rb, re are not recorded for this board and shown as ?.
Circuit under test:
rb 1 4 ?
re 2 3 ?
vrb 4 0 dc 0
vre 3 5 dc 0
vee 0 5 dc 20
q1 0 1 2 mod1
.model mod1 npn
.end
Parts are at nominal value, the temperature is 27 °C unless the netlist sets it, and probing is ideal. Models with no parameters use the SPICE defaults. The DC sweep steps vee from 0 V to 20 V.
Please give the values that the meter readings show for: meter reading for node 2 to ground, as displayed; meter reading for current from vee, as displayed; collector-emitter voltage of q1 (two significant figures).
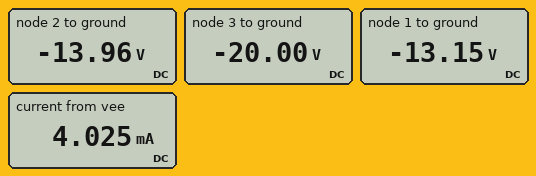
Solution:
-13.96 V
4.025 mA
14 V
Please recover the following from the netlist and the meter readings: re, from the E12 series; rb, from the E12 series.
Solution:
1.5 kΩ
330 kΩ
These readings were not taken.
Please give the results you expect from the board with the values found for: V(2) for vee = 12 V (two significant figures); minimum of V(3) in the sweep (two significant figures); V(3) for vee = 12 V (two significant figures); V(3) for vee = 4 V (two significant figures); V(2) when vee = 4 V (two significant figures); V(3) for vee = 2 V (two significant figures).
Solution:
-8.5 V
-20 V
-12 V
-4.0 V
-3.0 V
-2.0 V
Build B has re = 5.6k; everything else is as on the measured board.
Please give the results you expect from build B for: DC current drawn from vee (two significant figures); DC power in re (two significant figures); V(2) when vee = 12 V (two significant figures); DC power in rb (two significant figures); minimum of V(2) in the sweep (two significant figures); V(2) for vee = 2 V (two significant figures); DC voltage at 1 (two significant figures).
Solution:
2.2 mA
26 mW
-4.9 V
150 µW
-7.9 V
-1.2 V
-7.1 V
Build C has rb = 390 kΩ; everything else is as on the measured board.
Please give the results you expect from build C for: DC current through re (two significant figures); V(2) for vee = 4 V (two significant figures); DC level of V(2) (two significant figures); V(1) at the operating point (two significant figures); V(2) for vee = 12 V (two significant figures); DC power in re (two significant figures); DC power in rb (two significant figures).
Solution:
3.6 mA
-3.1 V
-15 V
-14 V
-8.9 V
19 mW
490 µW
